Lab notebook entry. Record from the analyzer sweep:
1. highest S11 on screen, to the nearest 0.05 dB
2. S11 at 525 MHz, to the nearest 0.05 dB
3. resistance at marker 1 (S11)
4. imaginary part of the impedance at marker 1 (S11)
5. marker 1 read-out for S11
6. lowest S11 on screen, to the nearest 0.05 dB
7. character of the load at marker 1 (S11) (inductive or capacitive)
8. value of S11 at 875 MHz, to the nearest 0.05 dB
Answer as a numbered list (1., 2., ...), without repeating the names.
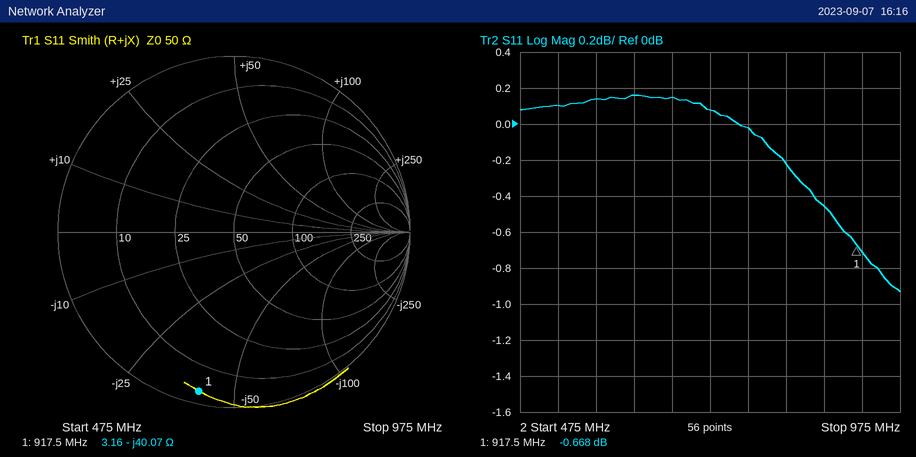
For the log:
1. 0.15 dB
2. 0.10 dB
3. 3.16 Ω
4. -40.07 Ω
5. -0.668 dB
6. -0.95 dB
7. capacitive
8. -0.45 dB
